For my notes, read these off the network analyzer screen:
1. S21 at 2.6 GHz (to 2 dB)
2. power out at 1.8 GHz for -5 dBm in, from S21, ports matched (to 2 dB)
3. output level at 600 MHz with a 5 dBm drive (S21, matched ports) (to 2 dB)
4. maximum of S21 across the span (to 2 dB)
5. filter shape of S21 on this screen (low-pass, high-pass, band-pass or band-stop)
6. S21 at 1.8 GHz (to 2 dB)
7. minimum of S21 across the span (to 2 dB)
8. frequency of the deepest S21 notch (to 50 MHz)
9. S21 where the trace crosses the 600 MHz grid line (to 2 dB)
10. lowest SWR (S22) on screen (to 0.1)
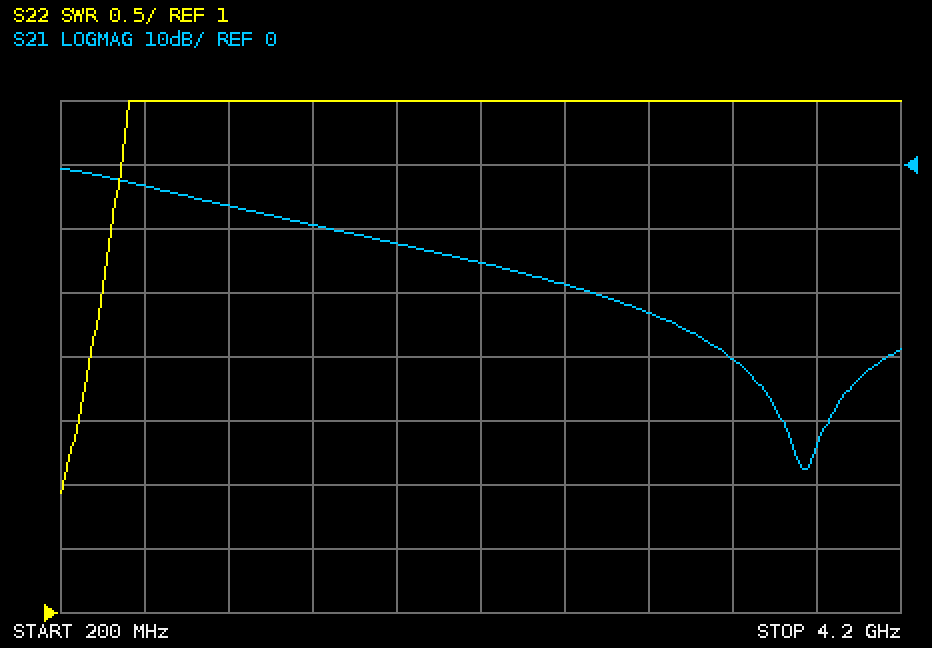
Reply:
-18 dB
-18 dBm
2 dBm
0 dB
low-pass
-12 dB
-48 dB
3.75 GHz
-4 dB
1.9
